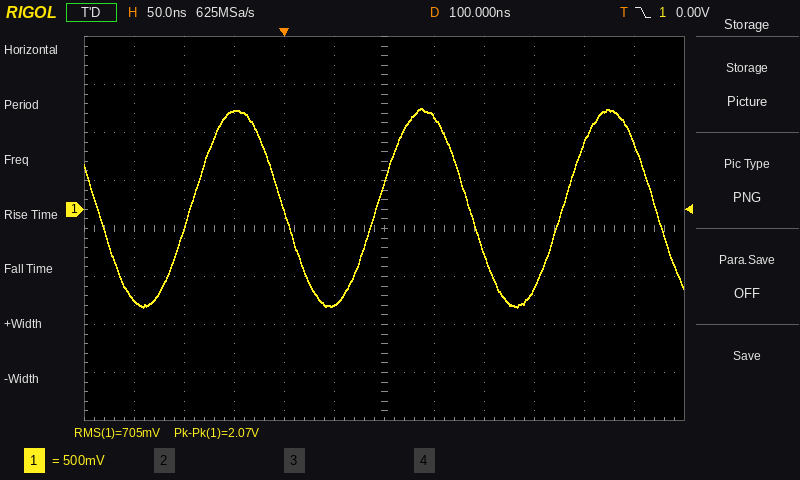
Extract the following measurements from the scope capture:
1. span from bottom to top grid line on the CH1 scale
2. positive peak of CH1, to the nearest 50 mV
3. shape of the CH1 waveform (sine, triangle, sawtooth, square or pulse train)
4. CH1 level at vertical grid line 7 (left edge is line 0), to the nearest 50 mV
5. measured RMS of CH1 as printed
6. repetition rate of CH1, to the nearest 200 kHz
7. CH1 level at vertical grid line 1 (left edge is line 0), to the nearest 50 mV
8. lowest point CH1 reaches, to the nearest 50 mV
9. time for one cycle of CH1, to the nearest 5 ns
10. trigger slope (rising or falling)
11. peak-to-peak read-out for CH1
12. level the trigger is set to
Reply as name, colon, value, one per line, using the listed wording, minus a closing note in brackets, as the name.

span from bottom to top grid line on the CH1 scale: 4 V
positive peak of CH1, to the nearest 50 mV: 1.05 V
shape of the CH1 waveform: sine
CH1 level at vertical grid line 7 (left edge is line 0), to the nearest 50 mV: 950 mV
measured RMS of CH1 as printed: 705 mV
repetition rate of CH1, to the nearest 200 kHz: 5.4 MHz
CH1 level at vertical grid line 1 (left edge is line 0), to the nearest 50 mV: -950 mV
lowest point CH1 reaches, to the nearest 50 mV: -1.00 V
time for one cycle of CH1, to the nearest 5 ns: 185 ns
trigger slope: falling
peak-to-peak read-out for CH1: 2.07 V
level the trigger is set to: 0.00 V
